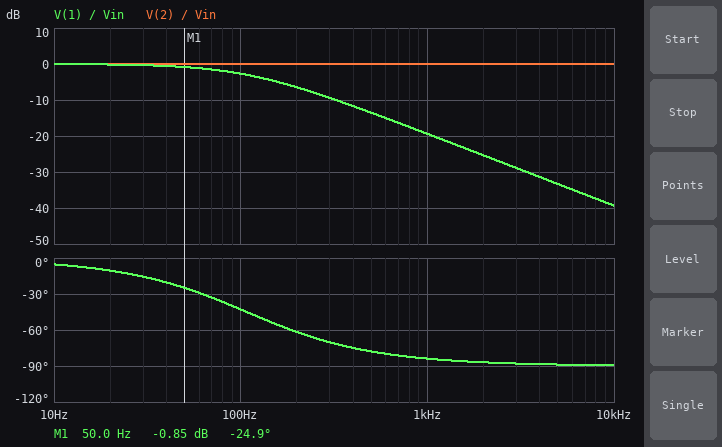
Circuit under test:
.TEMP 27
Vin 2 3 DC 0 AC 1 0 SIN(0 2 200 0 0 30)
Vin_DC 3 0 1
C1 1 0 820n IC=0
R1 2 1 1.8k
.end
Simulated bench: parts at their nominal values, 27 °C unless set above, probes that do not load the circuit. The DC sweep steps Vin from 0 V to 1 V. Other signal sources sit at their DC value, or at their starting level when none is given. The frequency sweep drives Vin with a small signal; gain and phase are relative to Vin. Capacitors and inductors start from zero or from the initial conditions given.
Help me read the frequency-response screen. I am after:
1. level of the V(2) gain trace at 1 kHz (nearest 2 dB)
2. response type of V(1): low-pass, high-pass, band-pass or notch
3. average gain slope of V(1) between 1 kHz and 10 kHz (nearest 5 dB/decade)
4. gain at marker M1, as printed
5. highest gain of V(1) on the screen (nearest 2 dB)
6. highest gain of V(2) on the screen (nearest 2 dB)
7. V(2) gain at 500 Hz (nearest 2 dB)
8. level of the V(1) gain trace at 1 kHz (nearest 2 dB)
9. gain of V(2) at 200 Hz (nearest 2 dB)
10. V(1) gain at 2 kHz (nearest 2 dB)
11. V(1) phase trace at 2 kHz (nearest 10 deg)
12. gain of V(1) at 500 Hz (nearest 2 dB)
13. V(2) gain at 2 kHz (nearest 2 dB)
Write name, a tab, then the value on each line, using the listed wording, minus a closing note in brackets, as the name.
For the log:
level of the V(2) gain trace at 1 kHz	0 dB
response type of V(1): low-pass, high-pass, band-pass or notch	low-pass
average gain slope of V(1) between 1 kHz and 10 kHz	-20 dB/decade
gain at marker M1, as printed	-0.85 dB
highest gain of V(1) on the screen	0 dB
highest gain of V(2) on the screen	0 dB
V(2) gain at 500 Hz	0 dB
level of the V(1) gain trace at 1 kHz	-20 dB
gain of V(2) at 200 Hz	0 dB
V(1) gain at 2 kHz	-26 dB
V(1) phase trace at 2 kHz	-90 deg
gain of V(1) at 500 Hz	-14 dB
V(2) gain at 2 kHz	0 dB
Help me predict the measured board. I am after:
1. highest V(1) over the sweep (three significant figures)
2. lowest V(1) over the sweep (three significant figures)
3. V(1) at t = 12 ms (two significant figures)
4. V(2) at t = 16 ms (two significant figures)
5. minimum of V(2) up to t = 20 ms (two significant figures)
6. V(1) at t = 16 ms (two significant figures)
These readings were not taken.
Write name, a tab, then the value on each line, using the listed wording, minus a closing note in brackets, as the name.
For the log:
highest V(1) over the sweep	2.00 V
lowest V(1) over the sweep	1.00 V
V(1) at t = 12 ms	1.9 V
V(2) at t = 16 ms	3.0 V
minimum of V(2) up to t = 20 ms	-1.0 V
V(1) at t = 16 ms	1.6 V
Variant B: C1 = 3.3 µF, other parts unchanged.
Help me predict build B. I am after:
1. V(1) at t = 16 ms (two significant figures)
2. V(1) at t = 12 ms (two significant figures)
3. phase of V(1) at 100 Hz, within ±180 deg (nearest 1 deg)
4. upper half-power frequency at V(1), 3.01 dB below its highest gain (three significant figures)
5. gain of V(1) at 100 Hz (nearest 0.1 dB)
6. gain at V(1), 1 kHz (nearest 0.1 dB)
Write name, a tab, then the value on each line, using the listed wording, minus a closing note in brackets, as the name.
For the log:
V(1) at t = 16 ms	1.0 V
V(1) at t = 12 ms	1.2 V
phase of V(1) at 100 Hz, within ±180 deg	-75 deg
upper half-power frequency at V(1), 3.01 dB below its highest gain	26.8 Hz
gain of V(1) at 100 Hz	-11.7 dB
gain at V(1), 1 kHz	-31.4 dB
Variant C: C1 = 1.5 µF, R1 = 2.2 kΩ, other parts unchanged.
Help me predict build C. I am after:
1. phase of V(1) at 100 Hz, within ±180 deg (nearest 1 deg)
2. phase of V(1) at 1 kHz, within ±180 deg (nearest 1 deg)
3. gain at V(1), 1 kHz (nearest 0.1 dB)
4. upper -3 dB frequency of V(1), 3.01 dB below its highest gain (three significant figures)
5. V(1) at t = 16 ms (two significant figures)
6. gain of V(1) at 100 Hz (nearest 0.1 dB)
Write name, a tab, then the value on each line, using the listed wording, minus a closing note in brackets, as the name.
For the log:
phase of V(1) at 100 Hz, within ±180 deg	-64 deg
phase of V(1) at 1 kHz, within ±180 deg	-87 deg
gain at V(1), 1 kHz	-26.3 dB
upper -3 dB frequency of V(1), 3.01 dB below its highest gain	48.2 Hz
V(1) at t = 16 ms	1.2 V
gain of V(1) at 100 Hz	-7.2 dB
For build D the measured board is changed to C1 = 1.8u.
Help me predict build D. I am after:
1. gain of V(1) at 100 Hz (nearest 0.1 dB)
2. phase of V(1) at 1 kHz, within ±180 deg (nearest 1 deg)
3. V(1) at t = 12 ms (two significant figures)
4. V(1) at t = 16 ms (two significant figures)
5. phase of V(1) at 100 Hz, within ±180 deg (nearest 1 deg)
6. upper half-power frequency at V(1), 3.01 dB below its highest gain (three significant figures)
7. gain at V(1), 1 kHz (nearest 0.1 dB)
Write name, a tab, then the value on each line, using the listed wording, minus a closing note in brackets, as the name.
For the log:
gain of V(1) at 100 Hz	-7.1 dB
phase of V(1) at 1 kHz, within ±180 deg	-87 deg
V(1) at t = 12 ms	1.5 V
V(1) at t = 16 ms	1.2 V
phase of V(1) at 100 Hz, within ±180 deg	-64 deg
upper half-power frequency at V(1), 3.01 dB below its highest gain	49.1 Hz
gain at V(1), 1 kHz	-26.2 dB
